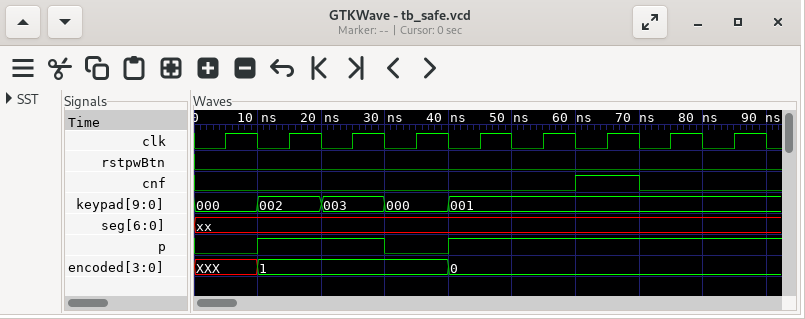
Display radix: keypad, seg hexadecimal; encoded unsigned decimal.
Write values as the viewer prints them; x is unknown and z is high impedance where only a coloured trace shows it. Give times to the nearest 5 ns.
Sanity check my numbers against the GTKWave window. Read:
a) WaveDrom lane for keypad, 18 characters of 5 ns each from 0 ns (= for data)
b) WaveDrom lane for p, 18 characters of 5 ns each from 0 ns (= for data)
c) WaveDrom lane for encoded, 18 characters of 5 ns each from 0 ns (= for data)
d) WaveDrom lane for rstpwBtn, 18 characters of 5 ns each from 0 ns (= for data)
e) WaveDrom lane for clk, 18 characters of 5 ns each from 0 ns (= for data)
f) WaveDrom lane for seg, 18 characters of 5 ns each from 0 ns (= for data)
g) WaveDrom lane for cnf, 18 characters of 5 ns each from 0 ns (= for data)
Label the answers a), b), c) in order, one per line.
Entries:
a) {name: 'keypad', wave: '=.=.=.=.=.........', data: '000 002 003 000 001'}
b) {name: 'p', wave: '0.1...0.1.........'}
c) {name: 'encoded', wave: 'x.=.....=.........', data: '1 0'}
d) {name: 'rstpwBtn', wave: '0.................'}
e) {name: 'clk', wave: '010101010101010101'}
f) {name: 'seg', wave: 'x.................'}
g) {name: 'cnf', wave: '0...........1.0...'}
